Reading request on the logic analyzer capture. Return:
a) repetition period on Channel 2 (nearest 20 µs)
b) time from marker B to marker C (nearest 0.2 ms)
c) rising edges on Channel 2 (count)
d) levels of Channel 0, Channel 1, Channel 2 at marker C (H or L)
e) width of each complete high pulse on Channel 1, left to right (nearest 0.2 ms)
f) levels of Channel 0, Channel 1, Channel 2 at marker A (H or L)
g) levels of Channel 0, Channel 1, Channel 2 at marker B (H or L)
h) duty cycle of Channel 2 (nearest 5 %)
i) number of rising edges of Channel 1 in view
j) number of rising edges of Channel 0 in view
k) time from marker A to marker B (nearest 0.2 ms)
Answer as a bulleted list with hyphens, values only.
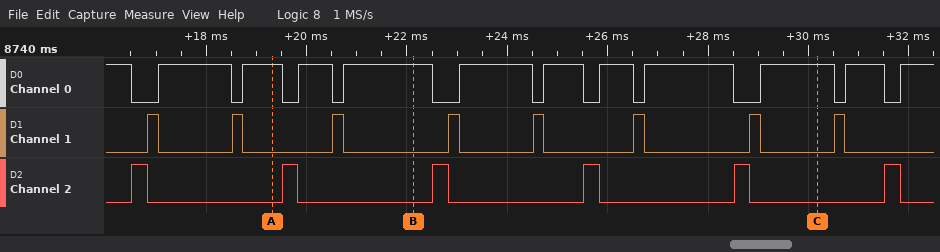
- 3000 µs
- 8 ms
- 6
- Channel 0=H, Channel 1=L, Channel 2=L
- 0.2 ms, 0.2 ms, 0.2 ms, 0.2 ms, 0.2 ms, 0.2 ms, 0.2 ms, 0.2 ms
- Channel 0=H, Channel 1=L, Channel 2=L
- Channel 0=H, Channel 1=L, Channel 2=L
- 10 %
- 8
- 11
- 2.8 ms
